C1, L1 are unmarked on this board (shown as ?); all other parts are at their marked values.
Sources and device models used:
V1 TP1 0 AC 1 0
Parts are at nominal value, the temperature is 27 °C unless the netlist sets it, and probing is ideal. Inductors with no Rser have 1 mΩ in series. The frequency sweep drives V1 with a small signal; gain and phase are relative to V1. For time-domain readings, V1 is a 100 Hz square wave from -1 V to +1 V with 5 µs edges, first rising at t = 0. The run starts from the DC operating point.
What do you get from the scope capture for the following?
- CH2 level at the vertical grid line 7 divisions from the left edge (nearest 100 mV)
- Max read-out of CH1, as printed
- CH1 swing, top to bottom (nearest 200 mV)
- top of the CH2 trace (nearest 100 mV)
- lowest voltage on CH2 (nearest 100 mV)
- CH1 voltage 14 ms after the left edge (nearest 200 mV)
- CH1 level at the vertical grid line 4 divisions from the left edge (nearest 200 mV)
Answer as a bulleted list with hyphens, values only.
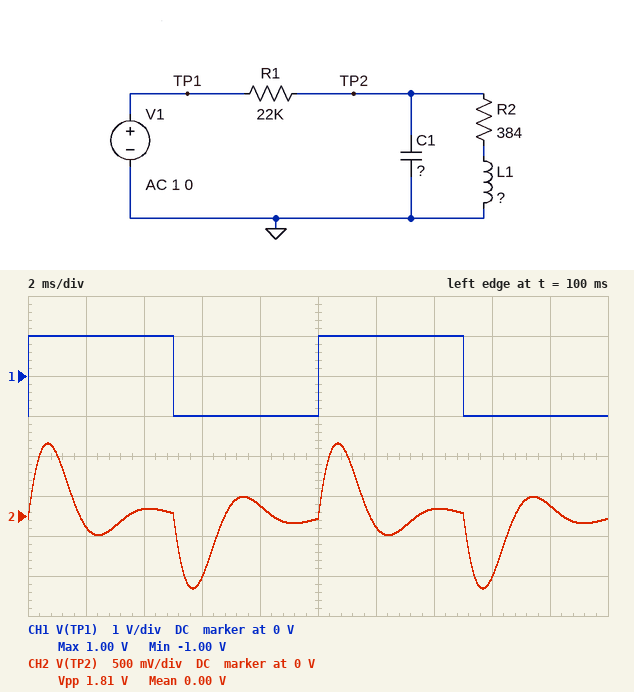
- 100 mV
- 1.00 V
- 2.0 V
- 900 mV
- -900 mV
- 1.0 V
- -1.0 V
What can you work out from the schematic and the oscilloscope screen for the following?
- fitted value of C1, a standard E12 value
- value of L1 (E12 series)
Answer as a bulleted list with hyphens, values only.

- 33 nF
- 8.2 H
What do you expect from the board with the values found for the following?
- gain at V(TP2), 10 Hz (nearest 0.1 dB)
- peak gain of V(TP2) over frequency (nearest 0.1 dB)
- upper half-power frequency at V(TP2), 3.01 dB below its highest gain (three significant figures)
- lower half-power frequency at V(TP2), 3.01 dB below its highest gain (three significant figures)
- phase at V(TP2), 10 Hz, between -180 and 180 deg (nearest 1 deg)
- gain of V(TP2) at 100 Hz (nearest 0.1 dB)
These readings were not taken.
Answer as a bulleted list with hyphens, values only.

- -30.8 dB
- -0.3 dB
- 442 Hz
- 215 Hz
- 52 deg
- -12.1 dB
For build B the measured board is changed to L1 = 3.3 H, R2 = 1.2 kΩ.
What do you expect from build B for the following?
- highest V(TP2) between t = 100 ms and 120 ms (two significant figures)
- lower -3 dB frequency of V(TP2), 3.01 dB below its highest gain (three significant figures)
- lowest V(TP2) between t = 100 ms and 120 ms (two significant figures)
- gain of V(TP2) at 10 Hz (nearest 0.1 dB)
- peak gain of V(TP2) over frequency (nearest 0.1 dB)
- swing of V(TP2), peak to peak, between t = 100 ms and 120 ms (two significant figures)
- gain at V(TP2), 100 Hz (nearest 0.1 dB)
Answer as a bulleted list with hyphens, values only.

- 630 mV
- 375 Hz
- -630 mV
- -25.6 dB
- -2.0 dB
- 1.3 V
- -19.4 dB
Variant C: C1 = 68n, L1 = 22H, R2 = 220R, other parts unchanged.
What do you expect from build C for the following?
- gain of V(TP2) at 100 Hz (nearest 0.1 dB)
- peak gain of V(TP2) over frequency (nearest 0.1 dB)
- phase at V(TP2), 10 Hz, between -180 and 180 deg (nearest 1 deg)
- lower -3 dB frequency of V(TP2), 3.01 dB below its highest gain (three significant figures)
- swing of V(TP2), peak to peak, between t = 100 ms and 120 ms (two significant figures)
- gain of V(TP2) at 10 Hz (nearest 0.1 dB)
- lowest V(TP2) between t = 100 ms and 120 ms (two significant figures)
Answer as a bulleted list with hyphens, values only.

- -1.7 dB
- -0.1 dB
- 77 deg
- 87.5 Hz
- 2.4 V
- -24.0 dB
- -1.2 V
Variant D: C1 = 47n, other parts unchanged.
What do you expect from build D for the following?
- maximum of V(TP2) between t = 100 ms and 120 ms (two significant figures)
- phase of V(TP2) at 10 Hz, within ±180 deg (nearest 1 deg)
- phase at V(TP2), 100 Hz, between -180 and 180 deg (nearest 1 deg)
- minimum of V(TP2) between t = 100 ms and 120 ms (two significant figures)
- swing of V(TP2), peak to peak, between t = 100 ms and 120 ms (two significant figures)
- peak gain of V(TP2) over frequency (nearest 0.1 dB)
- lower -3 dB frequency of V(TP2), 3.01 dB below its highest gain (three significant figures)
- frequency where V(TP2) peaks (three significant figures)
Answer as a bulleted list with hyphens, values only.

- 760 mV
- 52 deg
- 70 deg
- -760 mV
- 1.5 V
- -0.4 dB
- 190 Hz
- 259 Hz
